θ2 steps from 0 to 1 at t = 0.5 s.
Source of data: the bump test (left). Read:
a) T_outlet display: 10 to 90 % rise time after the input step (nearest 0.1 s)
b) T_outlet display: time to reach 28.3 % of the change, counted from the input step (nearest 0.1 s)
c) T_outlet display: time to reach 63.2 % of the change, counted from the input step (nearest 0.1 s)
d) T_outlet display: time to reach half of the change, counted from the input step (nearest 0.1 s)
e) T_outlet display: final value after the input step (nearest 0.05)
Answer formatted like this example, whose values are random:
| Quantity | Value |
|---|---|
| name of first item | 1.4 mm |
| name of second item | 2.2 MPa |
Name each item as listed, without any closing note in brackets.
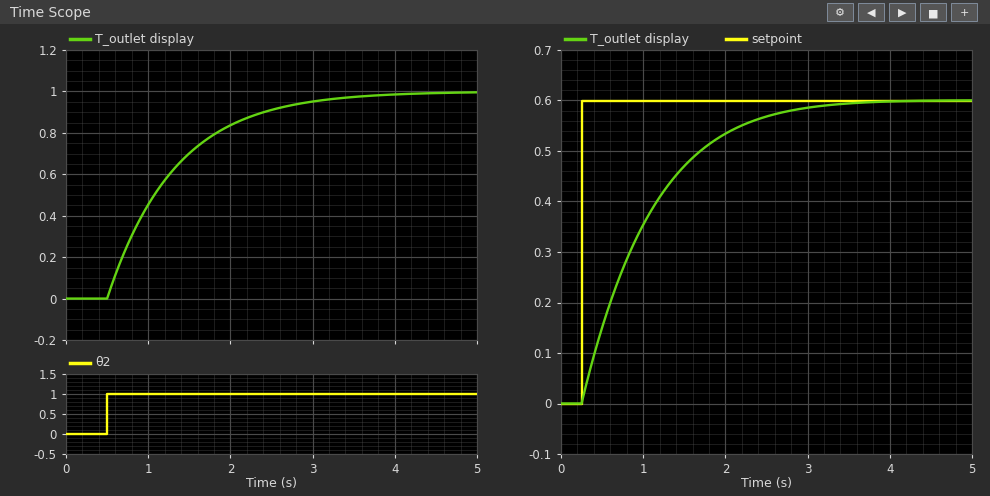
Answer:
| Quantity | Value |
|---|---|
| T_outlet display: 10 to 90 % rise time after the input step | 1.8 s |
| T_outlet display: time to reach 28.3 % of the change, counted from the input step | 0.3 s |
| T_outlet display: time to reach 63.2 % of the change, counted from the input step | 0.8 s |
| T_outlet display: time to reach half of the change, counted from the input step | 0.6 s |
| T_outlet display: final value after the input step | 1.00 |
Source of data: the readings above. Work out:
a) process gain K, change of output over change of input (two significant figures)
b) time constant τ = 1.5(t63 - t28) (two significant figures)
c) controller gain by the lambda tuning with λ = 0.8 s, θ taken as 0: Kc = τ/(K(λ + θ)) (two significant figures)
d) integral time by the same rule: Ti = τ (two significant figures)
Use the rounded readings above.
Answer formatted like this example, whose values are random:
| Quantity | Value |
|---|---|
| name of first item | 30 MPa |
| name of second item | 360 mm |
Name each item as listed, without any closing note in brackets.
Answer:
| Quantity | Value |
|---|---|
| process gain K, change of output over change of input | 1.0 |
| time constant τ = 1.5(t63 - t28) | 0.75 s |
| controller gain by the lambda tuning with λ = 0.8 s, θ taken as 0: Kc = τ/(K(λ + θ)) | 0.94 |
| integral time by the same rule: Ti = τ | 0.75 s |
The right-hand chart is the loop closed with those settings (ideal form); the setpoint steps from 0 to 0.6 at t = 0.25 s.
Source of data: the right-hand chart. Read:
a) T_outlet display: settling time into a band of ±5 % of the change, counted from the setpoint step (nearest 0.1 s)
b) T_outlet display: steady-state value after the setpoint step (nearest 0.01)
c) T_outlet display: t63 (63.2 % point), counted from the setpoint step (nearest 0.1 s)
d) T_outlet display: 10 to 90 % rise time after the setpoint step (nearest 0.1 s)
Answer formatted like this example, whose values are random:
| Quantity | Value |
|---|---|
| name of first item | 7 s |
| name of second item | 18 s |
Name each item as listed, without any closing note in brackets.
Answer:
| Quantity | Value |
|---|---|
| T_outlet display: settling time into a band of ±5 % of the change, counted from the setpoint step | 2.3 s |
| T_outlet display: steady-state value after the setpoint step | 0.60 |
| T_outlet display: t63 (63.2 % point), counted from the setpoint step | 0.8 s |
| T_outlet display: 10 to 90 % rise time after the setpoint step | 1.7 s |
